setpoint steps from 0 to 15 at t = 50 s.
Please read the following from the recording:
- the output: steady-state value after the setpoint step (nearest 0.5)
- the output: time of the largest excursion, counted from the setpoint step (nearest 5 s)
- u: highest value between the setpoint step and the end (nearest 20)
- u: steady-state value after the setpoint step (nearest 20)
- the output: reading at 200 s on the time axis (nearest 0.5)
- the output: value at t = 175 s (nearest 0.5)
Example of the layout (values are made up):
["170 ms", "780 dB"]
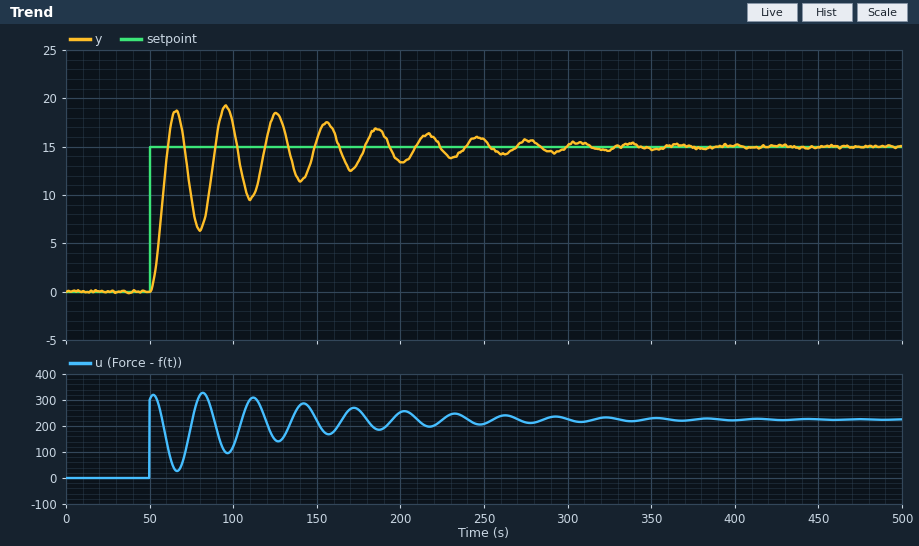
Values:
["15.0", "45 s", "320", "220", "13.5", "13.5"]
